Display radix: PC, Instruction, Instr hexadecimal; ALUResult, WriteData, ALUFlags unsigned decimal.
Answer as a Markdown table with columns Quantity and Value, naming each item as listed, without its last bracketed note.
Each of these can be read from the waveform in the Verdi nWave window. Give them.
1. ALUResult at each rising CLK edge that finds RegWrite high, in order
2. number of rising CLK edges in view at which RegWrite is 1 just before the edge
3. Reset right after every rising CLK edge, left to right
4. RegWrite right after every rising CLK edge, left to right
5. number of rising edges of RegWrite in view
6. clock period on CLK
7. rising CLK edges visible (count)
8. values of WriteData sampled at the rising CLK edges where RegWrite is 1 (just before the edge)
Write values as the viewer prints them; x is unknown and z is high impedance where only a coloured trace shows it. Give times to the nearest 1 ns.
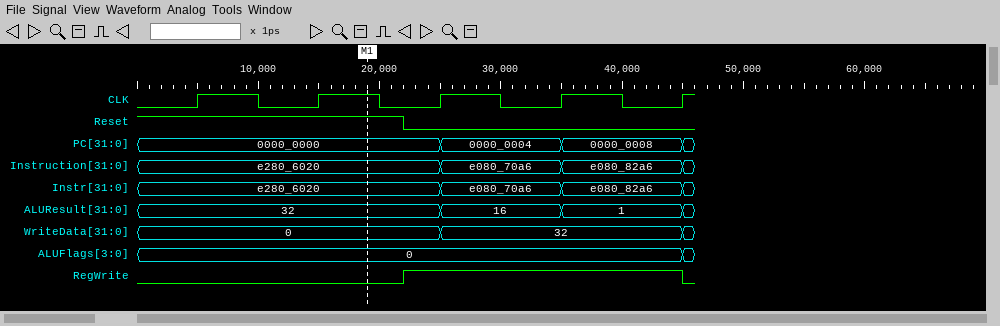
| Quantity | Value |
|---|---|
| ALUResult at each rising CLK edge that finds RegWrite high, in order | 32, 16, 1 |
| number of rising CLK edges in view at which RegWrite is 1 just before the edge | 3 |
| Reset right after every rising CLK edge, left to right | 1 1 0 0 0 |
| RegWrite right after every rising CLK edge, left to right | 0 0 1 1 0 |
| number of rising edges of RegWrite in view | 1 |
| clock period on CLK | 10 ns |
| rising CLK edges visible | 5 |
| values of WriteData sampled at the rising CLK edges where RegWrite is 1 | 0, 32, 32 |
